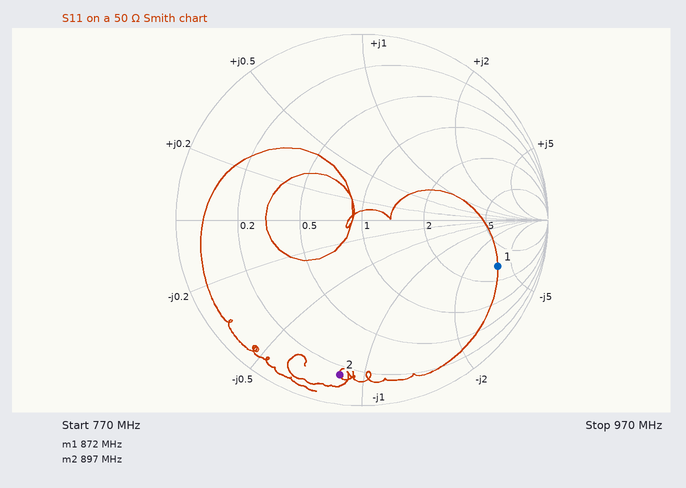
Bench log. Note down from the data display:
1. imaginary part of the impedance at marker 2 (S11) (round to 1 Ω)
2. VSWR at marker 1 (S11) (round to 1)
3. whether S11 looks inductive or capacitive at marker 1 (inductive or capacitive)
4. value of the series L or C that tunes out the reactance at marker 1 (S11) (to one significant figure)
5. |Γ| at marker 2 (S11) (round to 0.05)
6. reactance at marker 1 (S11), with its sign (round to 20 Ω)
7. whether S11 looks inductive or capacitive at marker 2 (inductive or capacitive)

-43 Ω
8
capacitive
30 nH
0.85
-180 Ω
capacitive
